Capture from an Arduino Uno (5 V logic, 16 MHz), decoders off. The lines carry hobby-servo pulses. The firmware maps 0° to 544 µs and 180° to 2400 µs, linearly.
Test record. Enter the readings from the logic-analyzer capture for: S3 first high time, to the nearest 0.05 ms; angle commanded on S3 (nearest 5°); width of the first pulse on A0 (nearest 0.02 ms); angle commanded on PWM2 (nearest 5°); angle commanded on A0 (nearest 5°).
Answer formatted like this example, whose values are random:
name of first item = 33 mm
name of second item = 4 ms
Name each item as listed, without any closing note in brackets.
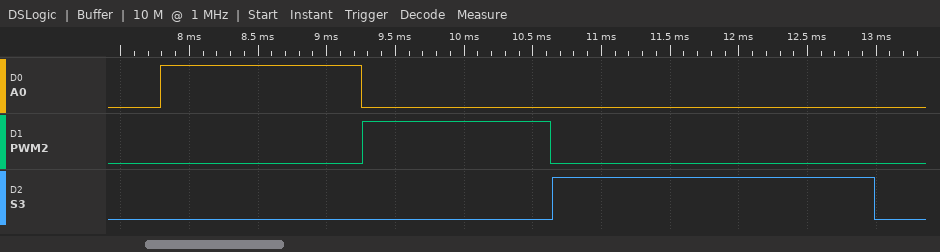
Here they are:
S3 first high time, to the nearest 0.05 ms = 2.35 ms
angle commanded on S3 = 175°
width of the first pulse on A0 = 1.46 ms
angle commanded on PWM2 = 80°
angle commanded on A0 = 90°
